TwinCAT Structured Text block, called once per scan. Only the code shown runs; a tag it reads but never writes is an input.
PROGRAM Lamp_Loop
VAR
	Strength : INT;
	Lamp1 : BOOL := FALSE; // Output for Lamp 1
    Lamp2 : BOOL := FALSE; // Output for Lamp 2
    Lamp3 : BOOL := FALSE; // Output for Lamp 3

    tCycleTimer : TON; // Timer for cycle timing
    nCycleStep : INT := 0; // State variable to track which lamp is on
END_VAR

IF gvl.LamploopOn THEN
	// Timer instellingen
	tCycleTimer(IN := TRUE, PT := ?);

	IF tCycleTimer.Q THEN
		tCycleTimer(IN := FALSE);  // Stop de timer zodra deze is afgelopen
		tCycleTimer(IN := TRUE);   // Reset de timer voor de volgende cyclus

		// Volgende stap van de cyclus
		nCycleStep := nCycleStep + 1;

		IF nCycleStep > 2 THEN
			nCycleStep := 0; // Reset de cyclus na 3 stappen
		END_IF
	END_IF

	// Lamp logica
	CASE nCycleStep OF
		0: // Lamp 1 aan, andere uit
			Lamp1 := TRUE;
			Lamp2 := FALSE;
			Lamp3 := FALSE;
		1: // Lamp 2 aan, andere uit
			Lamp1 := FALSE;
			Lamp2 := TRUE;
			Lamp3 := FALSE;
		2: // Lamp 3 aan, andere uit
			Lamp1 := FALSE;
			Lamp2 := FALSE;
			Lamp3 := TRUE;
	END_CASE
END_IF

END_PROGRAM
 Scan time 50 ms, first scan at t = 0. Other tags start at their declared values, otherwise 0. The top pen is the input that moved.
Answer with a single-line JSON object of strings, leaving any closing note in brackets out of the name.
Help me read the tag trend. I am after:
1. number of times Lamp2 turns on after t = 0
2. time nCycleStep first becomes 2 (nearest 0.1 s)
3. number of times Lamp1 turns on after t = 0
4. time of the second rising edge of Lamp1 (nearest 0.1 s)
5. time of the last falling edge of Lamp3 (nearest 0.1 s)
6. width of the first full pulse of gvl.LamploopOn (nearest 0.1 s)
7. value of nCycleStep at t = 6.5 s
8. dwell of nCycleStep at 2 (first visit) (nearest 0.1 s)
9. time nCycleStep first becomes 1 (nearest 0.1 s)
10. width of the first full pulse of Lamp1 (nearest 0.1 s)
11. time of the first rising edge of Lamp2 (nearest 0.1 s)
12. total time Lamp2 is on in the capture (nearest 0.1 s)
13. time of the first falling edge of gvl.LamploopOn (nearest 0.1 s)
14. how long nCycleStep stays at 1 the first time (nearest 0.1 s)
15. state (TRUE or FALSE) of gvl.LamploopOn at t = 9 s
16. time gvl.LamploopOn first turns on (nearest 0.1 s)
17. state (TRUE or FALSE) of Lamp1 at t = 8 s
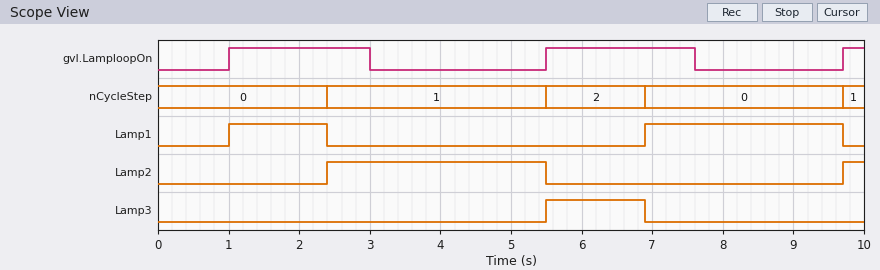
{"number of times Lamp2 turns on after t = 0": "2", "time nCycleStep first becomes 2": "5.5 s", "number of times Lamp1 turns on after t = 0": "2", "time of the second rising edge of Lamp1": "6.9 s", "time of the last falling edge of Lamp3": "6.9 s", "width of the first full pulse of gvl.LamploopOn": "2.0 s", "value of nCycleStep at t = 6.5 s": "2", "dwell of nCycleStep at 2 (first visit)": "1.4 s", "time nCycleStep first becomes 1": "2.4 s", "width of the first full pulse of Lamp1": "1.4 s", "time of the first rising edge of Lamp2": "2.4 s", "total time Lamp2 is on in the capture": "3.4 s", "time of the first falling edge of gvl.LamploopOn": "3.0 s", "how long nCycleStep stays at 1 the first time": "3.1 s", "state (TRUE or FALSE) of gvl.LamploopOn at t = 9 s": "FALSE", "time gvl.LamploopOn first turns on": "1.0 s", "state (TRUE or FALSE) of Lamp1 at t = 8 s": "TRUE"}
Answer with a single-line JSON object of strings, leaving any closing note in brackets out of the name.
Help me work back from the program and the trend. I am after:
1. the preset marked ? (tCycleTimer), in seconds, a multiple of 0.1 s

{"the preset marked ? (tCycleTimer), in seconds, a multiple of 0.1 s": "1.4 s"}
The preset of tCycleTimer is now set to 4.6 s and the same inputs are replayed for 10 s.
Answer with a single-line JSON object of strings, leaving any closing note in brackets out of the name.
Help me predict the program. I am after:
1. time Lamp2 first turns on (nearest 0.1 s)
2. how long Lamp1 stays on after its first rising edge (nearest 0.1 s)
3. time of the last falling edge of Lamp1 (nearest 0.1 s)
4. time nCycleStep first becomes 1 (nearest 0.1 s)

{"time Lamp2 first turns on": "5.6 s", "how long Lamp1 stays on after its first rising edge": "4.6 s", "time of the last falling edge of Lamp1": "5.6 s", "time nCycleStep first becomes 1": "5.6 s"}
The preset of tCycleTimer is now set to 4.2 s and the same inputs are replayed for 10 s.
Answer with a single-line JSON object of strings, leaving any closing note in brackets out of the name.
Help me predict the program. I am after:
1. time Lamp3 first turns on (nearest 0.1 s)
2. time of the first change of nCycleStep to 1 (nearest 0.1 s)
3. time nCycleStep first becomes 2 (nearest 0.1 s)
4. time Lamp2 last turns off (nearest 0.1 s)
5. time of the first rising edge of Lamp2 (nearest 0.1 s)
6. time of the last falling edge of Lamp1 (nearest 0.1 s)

{"time Lamp3 first turns on": "9.7 s", "time of the first change of nCycleStep to 1": "5.5 s", "time nCycleStep first becomes 2": "9.7 s", "time Lamp2 last turns off": "9.7 s", "time of the first rising edge of Lamp2": "5.5 s", "time of the last falling edge of Lamp1": "5.5 s"}
